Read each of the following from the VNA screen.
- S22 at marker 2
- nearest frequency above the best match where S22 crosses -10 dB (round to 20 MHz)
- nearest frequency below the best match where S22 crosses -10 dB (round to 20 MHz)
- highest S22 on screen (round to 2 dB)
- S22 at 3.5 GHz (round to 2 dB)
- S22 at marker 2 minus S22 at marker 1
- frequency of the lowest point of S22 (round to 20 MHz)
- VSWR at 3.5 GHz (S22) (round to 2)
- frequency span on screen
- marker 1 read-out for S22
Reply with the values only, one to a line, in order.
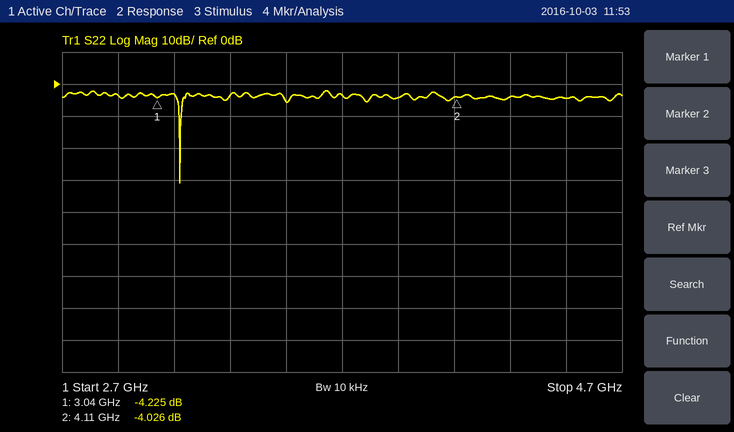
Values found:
-4.026 dB
3.12 GHz
3.12 GHz
-2 dB
-6 dB
0.199 dB
3.12 GHz
4
2 GHz
-4.225 dB
